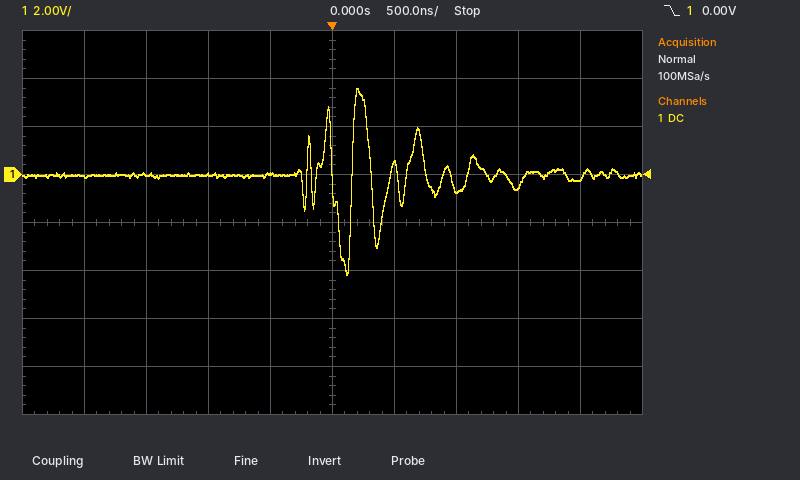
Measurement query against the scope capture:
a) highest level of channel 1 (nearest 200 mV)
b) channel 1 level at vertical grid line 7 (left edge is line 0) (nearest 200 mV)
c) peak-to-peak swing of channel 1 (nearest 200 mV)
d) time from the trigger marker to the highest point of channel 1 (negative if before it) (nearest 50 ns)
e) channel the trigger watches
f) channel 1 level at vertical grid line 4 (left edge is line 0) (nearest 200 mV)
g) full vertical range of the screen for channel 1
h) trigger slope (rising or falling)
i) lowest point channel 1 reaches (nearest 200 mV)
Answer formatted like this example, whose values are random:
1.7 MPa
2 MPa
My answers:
3.6 V
-600 mV
7.8 V
+200 ns
channel 1
0.0 V
16 V
falling
-4.2 V
